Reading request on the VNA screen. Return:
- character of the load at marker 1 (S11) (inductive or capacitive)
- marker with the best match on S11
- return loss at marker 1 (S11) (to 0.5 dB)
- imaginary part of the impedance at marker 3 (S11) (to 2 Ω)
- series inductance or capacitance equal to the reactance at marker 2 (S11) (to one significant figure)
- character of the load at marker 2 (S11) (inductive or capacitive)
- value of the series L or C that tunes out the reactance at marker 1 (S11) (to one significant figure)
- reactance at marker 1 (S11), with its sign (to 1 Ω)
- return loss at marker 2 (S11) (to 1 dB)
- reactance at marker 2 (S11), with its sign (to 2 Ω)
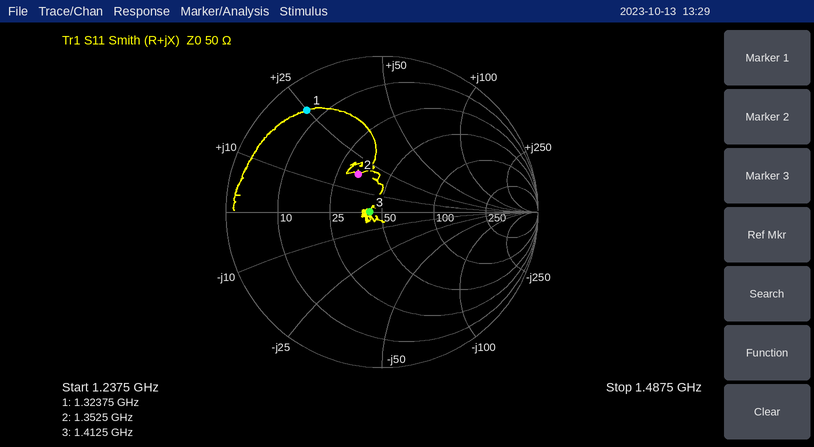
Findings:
inductive
marker 3
2.0 dB
0 Ω
2 nH
inductive
5 pF
+25 Ω
11 dB
+18 Ω
